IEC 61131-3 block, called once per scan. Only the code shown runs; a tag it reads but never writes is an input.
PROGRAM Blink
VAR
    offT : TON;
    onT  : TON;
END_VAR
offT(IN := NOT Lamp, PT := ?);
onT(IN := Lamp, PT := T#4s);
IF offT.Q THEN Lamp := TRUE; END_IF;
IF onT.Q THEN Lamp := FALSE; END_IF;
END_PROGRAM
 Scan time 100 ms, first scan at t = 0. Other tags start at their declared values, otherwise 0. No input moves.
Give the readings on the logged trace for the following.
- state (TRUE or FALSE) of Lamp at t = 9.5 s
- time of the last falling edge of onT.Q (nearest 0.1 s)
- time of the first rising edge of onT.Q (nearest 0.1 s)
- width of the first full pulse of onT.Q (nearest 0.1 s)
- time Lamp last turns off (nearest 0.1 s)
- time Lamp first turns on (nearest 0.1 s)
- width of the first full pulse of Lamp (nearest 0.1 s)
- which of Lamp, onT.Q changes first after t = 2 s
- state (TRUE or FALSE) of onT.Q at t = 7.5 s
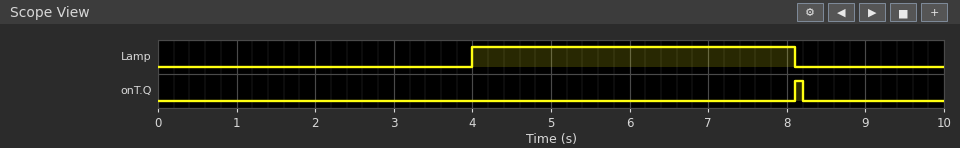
FALSE
8.2 s
8.1 s
0.1 s
8.1 s
4.0 s
4.1 s
Lamp
FALSE
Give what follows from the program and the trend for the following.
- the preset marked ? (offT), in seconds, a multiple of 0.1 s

4.0 s
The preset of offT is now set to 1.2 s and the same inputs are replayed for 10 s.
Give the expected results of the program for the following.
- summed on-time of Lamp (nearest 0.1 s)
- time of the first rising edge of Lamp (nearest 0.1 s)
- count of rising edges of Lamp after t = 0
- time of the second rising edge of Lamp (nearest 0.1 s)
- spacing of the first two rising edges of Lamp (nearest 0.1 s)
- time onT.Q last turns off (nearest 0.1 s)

7.5 s
1.2 s
2
6.6 s
5.4 s
5.4 s
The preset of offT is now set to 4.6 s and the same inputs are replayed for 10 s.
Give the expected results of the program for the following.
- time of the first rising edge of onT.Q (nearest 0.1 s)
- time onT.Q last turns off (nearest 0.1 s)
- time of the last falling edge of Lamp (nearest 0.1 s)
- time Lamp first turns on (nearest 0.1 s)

8.7 s
8.8 s
8.7 s
4.6 s
